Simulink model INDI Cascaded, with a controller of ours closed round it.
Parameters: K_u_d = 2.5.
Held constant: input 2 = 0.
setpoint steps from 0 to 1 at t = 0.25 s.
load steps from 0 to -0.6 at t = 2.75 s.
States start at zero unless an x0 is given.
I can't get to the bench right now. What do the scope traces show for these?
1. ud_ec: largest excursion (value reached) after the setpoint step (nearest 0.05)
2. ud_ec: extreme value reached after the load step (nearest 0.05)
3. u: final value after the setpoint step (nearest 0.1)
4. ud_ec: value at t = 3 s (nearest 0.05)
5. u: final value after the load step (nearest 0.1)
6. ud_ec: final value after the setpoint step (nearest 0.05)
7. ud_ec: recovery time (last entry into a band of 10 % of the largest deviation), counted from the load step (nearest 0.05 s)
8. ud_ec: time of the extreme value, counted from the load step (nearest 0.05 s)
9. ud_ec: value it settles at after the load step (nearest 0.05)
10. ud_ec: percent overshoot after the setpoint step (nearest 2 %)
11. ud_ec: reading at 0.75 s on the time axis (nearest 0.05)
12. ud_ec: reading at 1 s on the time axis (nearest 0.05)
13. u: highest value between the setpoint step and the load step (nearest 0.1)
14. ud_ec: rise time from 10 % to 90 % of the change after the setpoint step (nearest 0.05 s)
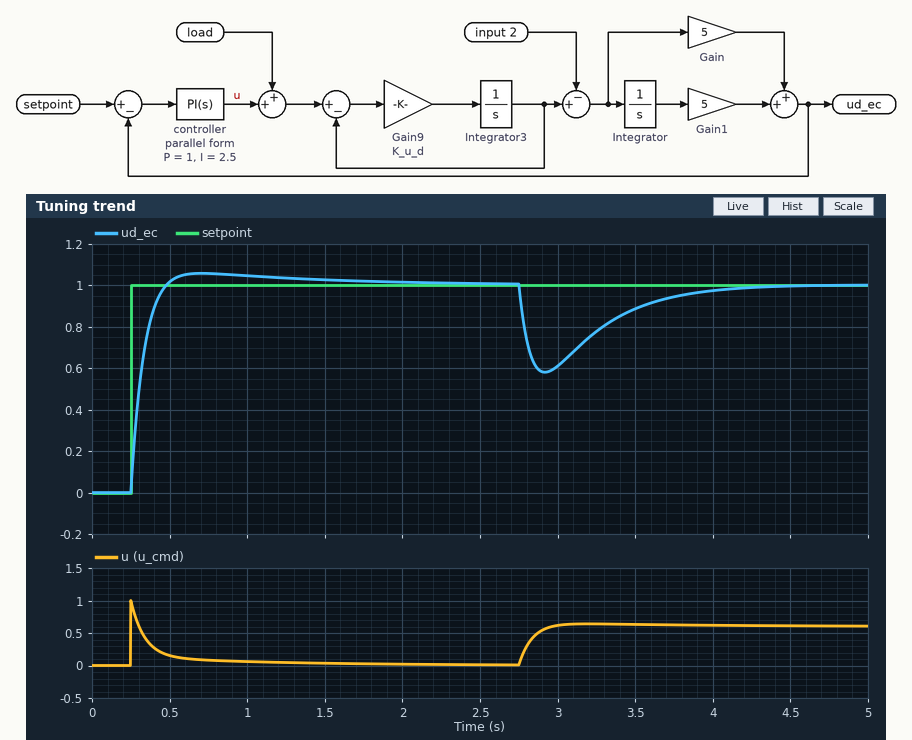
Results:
1.05
0.60
0.0
0.60
0.6
1.00
1.10 s
0.15 s
1.00
6 %
1.05
1.05
1.0
0.15 s
